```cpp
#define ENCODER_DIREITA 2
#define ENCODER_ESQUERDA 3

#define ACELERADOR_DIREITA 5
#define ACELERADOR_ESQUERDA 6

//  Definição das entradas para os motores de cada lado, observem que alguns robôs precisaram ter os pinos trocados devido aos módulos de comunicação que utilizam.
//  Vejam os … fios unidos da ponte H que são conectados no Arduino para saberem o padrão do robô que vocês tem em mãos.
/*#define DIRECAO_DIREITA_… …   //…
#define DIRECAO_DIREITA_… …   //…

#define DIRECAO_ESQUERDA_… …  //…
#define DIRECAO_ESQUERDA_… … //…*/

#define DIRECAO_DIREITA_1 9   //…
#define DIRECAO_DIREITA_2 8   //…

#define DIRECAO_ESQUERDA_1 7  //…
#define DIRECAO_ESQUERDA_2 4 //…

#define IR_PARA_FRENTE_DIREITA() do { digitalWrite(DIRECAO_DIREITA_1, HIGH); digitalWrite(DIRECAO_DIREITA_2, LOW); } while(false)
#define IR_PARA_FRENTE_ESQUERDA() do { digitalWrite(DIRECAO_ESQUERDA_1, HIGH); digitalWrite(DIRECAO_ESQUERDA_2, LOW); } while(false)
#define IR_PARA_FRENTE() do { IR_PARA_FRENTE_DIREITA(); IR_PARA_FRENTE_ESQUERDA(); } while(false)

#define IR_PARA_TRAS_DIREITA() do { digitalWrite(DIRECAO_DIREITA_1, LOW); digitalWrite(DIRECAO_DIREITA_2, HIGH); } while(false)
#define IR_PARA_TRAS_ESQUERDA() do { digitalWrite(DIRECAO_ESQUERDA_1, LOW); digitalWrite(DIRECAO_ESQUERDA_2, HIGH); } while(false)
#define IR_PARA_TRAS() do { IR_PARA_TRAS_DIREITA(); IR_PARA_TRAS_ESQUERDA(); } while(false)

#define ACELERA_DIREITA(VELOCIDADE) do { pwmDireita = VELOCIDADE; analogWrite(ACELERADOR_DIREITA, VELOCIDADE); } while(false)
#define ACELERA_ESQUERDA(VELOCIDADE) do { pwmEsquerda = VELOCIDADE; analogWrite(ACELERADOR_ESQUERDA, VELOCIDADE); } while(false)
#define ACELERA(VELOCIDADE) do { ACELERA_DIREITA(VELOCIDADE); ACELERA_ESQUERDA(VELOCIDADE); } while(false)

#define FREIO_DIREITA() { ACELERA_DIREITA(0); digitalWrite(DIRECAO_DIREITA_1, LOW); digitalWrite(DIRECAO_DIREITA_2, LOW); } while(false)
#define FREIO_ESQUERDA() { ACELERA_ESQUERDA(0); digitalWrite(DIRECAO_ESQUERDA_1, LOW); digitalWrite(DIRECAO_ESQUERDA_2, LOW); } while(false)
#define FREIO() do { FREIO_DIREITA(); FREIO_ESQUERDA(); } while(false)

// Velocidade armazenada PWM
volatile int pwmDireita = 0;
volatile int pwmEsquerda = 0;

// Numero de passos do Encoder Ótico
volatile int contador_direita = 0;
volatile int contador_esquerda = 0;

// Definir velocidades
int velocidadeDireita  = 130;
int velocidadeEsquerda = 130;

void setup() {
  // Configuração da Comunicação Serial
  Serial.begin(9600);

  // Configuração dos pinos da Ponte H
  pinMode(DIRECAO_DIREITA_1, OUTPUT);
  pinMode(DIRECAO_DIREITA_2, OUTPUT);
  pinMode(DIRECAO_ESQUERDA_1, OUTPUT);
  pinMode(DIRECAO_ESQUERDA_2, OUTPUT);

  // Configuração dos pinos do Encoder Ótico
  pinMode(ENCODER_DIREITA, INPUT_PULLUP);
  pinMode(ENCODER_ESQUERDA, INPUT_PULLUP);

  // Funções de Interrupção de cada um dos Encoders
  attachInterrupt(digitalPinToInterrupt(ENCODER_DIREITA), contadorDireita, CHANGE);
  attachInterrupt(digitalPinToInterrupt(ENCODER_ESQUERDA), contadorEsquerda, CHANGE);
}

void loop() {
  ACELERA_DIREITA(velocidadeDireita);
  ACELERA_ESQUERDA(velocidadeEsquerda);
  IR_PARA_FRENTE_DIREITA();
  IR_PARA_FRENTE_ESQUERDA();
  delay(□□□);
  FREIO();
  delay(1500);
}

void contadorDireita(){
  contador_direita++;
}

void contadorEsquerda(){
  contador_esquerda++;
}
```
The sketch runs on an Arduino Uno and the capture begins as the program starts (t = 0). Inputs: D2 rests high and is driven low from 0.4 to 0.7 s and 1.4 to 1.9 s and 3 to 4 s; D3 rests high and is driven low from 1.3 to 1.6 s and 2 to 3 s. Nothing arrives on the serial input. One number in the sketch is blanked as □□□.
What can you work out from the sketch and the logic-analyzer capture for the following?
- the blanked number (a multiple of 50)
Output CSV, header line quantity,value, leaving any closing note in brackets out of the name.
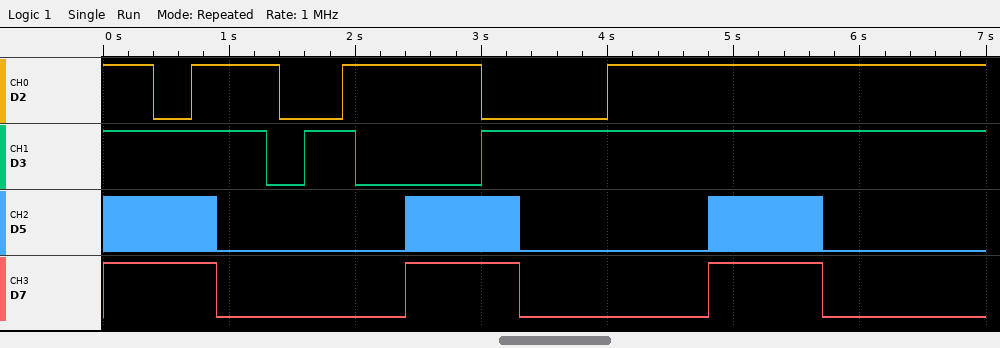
quantity,value
the blanked number,900
